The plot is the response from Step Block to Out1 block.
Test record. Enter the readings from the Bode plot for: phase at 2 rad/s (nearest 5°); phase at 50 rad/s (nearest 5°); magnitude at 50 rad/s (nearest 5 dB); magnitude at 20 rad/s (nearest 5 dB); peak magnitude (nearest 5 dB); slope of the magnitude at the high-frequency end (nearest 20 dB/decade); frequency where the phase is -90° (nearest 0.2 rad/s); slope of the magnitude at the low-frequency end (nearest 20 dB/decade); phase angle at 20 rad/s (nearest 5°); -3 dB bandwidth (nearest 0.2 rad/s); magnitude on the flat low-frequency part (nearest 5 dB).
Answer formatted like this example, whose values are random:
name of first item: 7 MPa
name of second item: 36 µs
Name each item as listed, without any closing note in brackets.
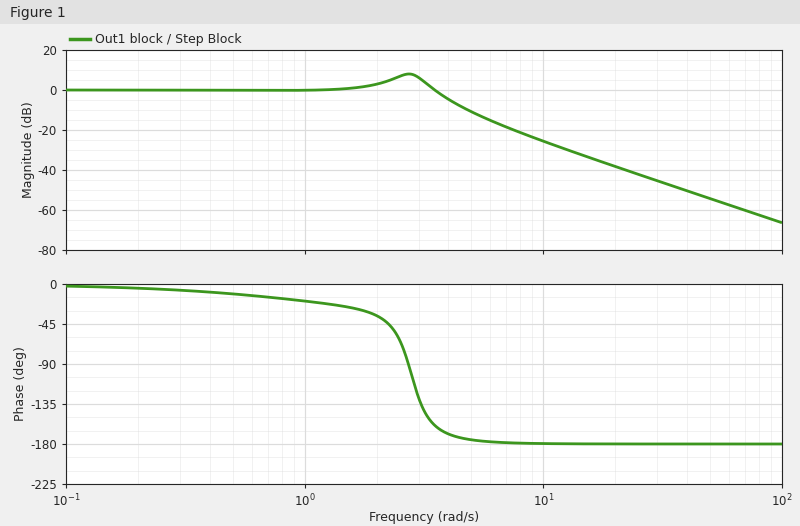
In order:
phase at 2 rad/s: -35°
phase at 50 rad/s: -180°
magnitude at 50 rad/s: -55 dB
magnitude at 20 rad/s: -40 dB
peak magnitude: 10 dB
slope of the magnitude at the high-frequency end: -40 dB/decade
frequency where the phase is -90°: 2.8 rad/s
slope of the magnitude at the low-frequency end: 0 dB/decade
phase angle at 20 rad/s: -180°
-3 dB bandwidth: 3.8 rad/s
magnitude on the flat low-frequency part: 0 dB
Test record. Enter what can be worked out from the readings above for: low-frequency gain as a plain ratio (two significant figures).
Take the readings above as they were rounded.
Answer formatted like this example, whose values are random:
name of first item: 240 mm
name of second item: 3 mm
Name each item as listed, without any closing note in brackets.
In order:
low-frequency gain as a plain ratio: 1.0
